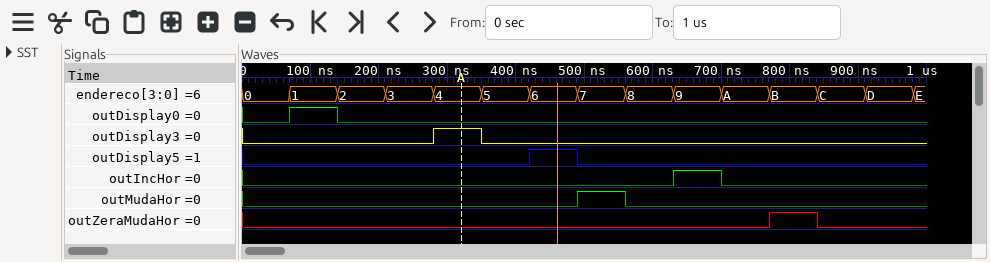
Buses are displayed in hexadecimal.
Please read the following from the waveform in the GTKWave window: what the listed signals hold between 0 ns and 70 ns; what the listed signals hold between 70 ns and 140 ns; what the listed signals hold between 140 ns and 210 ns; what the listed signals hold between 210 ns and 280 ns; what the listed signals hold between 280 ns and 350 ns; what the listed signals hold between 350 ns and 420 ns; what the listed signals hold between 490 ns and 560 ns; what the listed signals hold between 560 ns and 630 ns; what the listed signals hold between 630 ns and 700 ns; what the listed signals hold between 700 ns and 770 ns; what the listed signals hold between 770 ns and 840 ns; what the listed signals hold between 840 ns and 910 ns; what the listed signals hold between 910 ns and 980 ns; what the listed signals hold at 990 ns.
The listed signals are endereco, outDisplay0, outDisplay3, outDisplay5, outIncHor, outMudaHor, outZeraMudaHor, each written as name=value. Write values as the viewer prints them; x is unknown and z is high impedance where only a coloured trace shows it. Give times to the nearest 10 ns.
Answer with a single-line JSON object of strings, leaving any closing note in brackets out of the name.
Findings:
{"what the listed signals hold between 0 ns and 70 ns": "endereco=0, outDisplay0=0, outDisplay3=0, outDisplay5=0, outIncHor=0, outMudaHor=0, outZeraMudaHor=0", "what the listed signals hold between 70 ns and 140 ns": "endereco=1, outDisplay0=1, outDisplay3=0, outDisplay5=0, outIncHor=0, outMudaHor=0, outZeraMudaHor=0", "what the listed signals hold between 140 ns and 210 ns": "endereco=2, outDisplay0=0, outDisplay3=0, outDisplay5=0, outIncHor=0, outMudaHor=0, outZeraMudaHor=0", "what the listed signals hold between 210 ns and 280 ns": "endereco=3, outDisplay0=0, outDisplay3=0, outDisplay5=0, outIncHor=0, outMudaHor=0, outZeraMudaHor=0", "what the listed signals hold between 280 ns and 350 ns": "endereco=4, outDisplay0=0, outDisplay3=1, outDisplay5=0, outIncHor=0, outMudaHor=0, outZeraMudaHor=0", "what the listed signals hold between 350 ns and 420 ns": "endereco=5, outDisplay0=0, outDisplay3=0, outDisplay5=0, outIncHor=0, outMudaHor=0, outZeraMudaHor=0", "what the listed signals hold between 490 ns and 560 ns": "endereco=7, outDisplay0=0, outDisplay3=0, outDisplay5=0, outIncHor=0, outMudaHor=1, outZeraMudaHor=0", "what the listed signals hold between 560 ns and 630 ns": "endereco=8, outDisplay0=0, outDisplay3=0, outDisplay5=0, outIncHor=0, outMudaHor=0, outZeraMudaHor=0", "what the listed signals hold between 630 ns and 700 ns": "endereco=9, outDisplay0=0, outDisplay3=0, outDisplay5=0, outIncHor=1, outMudaHor=0, outZeraMudaHor=0", "what the listed signals hold between 700 ns and 770 ns": "endereco=A, outDisplay0=0, outDisplay3=0, outDisplay5=0, outIncHor=0, outMudaHor=0, outZeraMudaHor=0", "what the listed signals hold between 770 ns and 840 ns": "endereco=B, outDisplay0=0, outDisplay3=0, outDisplay5=0, outIncHor=0, outMudaHor=0, outZeraMudaHor=1", "what the listed signals hold between 840 ns and 910 ns": "endereco=C, outDisplay0=0, outDisplay3=0, outDisplay5=0, outIncHor=0, outMudaHor=0, outZeraMudaHor=0", "what the listed signals hold between 910 ns and 980 ns": "endereco=D, outDisplay0=0, outDisplay3=0, outDisplay5=0, outIncHor=0, outMudaHor=0, outZeraMudaHor=0", "what the listed signals hold at 990 ns": "endereco=E, outDisplay0=0, outDisplay3=0, outDisplay5=0, outIncHor=0, outMudaHor=0, outZeraMudaHor=0"}
